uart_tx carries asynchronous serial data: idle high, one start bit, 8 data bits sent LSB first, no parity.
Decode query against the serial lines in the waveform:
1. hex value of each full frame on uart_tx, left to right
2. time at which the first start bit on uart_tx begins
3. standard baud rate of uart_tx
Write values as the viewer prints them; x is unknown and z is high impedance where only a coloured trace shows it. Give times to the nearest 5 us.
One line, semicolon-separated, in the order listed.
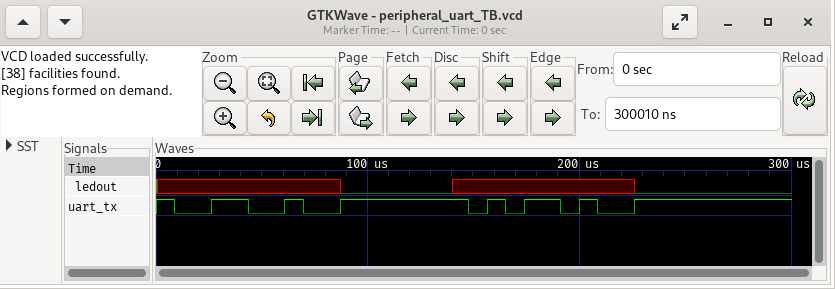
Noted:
26, 2D; 10 us; 115200 baud
